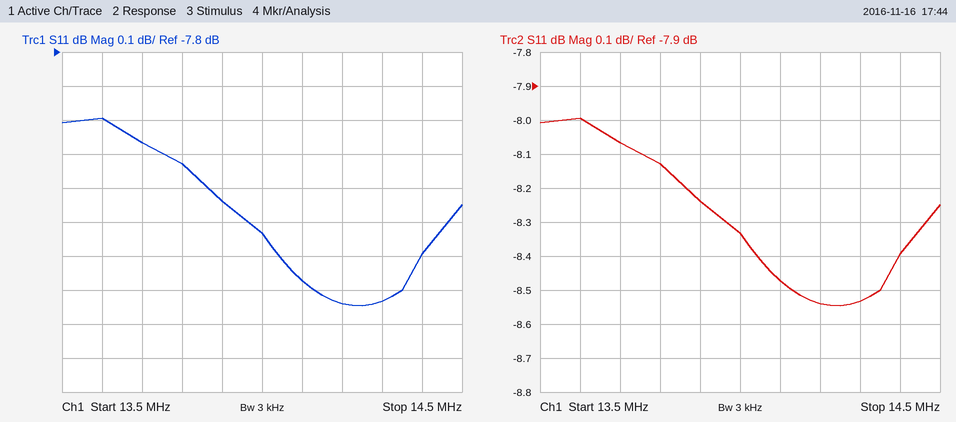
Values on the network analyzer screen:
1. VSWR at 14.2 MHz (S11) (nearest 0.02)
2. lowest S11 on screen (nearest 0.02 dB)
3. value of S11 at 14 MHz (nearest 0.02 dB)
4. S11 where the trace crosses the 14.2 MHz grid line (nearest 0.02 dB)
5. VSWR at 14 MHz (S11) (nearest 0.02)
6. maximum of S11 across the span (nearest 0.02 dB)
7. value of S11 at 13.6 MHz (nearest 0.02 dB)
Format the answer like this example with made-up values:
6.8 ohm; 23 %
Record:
2.20; -8.54 dB; -8.34 dB; -8.54 dB; 2.24; -8.00 dB; -8.00 dB
